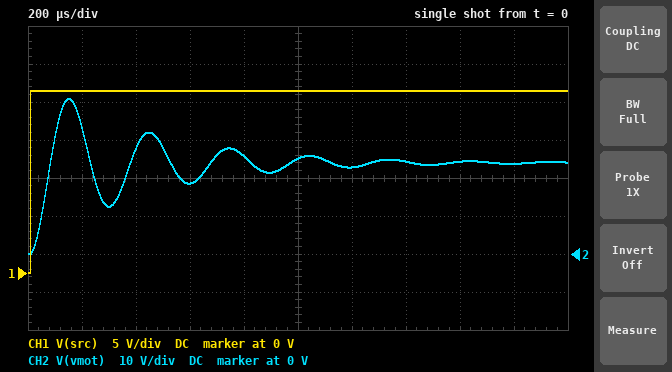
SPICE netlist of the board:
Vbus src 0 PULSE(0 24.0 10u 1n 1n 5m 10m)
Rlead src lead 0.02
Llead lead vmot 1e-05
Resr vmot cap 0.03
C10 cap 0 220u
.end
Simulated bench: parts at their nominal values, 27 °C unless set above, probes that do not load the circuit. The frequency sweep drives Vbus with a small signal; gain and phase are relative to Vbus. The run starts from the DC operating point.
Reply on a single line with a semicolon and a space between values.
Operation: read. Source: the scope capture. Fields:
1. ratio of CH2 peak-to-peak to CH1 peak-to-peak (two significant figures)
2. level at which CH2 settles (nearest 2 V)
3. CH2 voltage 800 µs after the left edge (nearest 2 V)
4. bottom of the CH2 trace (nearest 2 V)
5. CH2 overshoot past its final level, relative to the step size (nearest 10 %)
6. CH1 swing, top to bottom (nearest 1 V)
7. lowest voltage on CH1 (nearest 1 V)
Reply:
1.7; 24 V; 26 V; 0 V; 70 %; 24 V; 0 V
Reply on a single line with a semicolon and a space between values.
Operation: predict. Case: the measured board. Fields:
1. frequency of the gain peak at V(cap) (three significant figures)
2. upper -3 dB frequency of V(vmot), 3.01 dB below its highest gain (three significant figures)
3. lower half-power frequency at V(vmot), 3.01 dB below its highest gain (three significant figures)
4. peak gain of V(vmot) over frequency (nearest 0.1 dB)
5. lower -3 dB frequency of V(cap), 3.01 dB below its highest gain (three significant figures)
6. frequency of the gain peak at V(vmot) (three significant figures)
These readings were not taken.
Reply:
3.35 kHz; 3.73 kHz; 2.92 kHz; 12.7 dB; 2.92 kHz; 3.35 kHz
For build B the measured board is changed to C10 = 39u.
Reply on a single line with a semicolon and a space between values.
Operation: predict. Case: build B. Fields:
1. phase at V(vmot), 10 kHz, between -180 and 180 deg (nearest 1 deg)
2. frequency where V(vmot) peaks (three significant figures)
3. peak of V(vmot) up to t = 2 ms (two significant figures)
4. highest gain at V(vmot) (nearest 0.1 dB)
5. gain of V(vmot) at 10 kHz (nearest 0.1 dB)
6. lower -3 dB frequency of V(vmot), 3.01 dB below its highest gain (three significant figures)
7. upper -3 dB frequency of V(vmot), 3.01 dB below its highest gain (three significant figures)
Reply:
-163 deg; 8.04 kHz; 45 V; 20.1 dB; 5.2 dB; 7.63 kHz; 8.43 kHz
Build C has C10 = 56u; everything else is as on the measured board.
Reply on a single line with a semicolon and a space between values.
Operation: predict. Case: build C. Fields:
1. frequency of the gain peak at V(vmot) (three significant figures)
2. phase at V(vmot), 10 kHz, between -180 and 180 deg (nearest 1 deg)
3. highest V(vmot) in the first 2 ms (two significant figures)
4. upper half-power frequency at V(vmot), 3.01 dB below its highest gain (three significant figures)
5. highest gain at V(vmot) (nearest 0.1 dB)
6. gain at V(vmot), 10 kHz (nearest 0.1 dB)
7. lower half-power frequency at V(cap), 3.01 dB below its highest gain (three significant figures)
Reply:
6.70 kHz; -166 deg; 44 V; 7.09 kHz; 18.6 dB; -1.7 dB; 6.29 kHz
